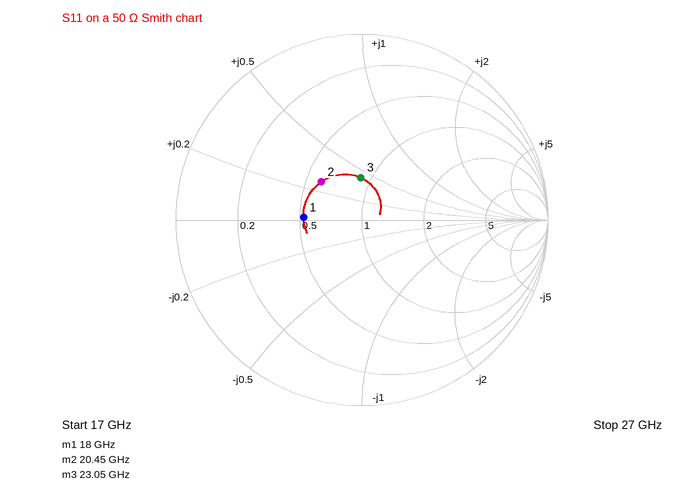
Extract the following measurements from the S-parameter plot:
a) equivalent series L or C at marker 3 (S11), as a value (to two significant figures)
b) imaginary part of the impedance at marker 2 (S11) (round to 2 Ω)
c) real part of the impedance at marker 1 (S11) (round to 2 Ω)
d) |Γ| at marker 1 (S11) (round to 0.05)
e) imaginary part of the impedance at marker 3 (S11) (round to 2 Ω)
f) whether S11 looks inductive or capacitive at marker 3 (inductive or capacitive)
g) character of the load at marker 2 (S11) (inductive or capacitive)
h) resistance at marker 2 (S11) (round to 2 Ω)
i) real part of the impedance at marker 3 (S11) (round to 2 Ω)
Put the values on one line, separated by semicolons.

150 pH; +14 Ω; 26 Ω; 0.30; +22 Ω; inductive; inductive; 30 Ω; 44 Ω
